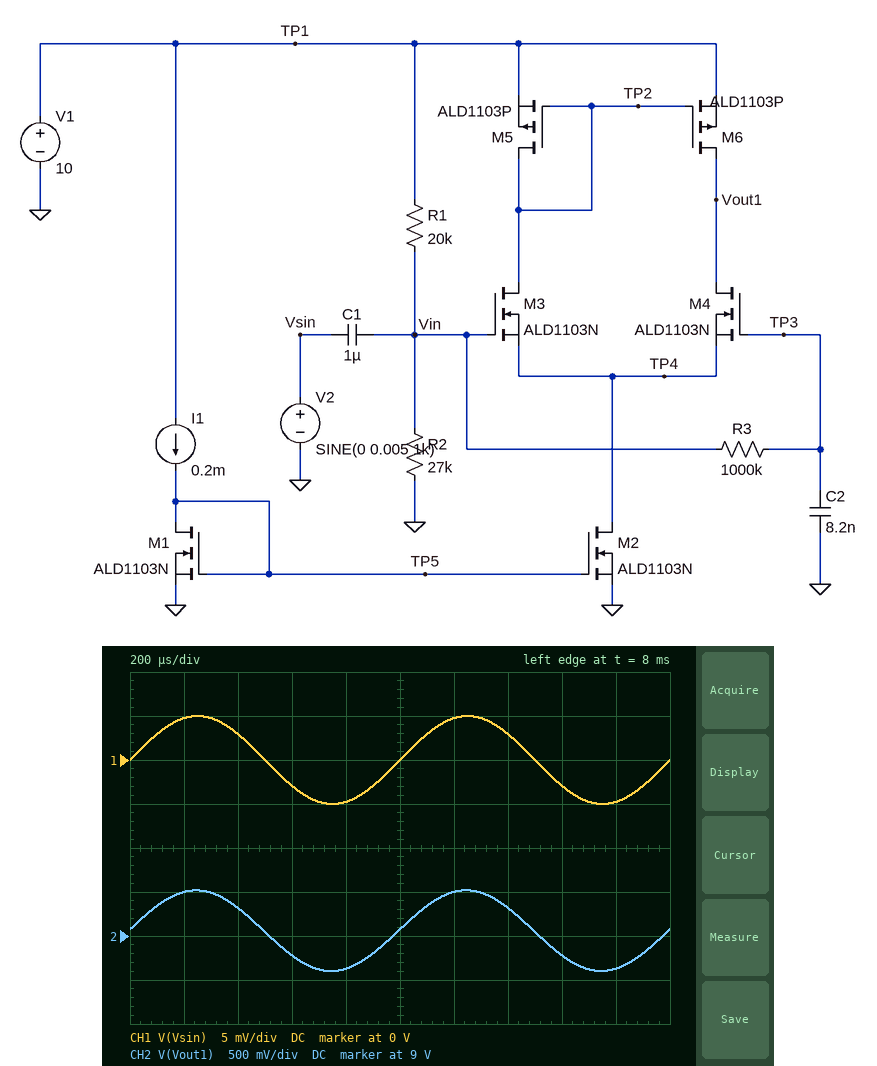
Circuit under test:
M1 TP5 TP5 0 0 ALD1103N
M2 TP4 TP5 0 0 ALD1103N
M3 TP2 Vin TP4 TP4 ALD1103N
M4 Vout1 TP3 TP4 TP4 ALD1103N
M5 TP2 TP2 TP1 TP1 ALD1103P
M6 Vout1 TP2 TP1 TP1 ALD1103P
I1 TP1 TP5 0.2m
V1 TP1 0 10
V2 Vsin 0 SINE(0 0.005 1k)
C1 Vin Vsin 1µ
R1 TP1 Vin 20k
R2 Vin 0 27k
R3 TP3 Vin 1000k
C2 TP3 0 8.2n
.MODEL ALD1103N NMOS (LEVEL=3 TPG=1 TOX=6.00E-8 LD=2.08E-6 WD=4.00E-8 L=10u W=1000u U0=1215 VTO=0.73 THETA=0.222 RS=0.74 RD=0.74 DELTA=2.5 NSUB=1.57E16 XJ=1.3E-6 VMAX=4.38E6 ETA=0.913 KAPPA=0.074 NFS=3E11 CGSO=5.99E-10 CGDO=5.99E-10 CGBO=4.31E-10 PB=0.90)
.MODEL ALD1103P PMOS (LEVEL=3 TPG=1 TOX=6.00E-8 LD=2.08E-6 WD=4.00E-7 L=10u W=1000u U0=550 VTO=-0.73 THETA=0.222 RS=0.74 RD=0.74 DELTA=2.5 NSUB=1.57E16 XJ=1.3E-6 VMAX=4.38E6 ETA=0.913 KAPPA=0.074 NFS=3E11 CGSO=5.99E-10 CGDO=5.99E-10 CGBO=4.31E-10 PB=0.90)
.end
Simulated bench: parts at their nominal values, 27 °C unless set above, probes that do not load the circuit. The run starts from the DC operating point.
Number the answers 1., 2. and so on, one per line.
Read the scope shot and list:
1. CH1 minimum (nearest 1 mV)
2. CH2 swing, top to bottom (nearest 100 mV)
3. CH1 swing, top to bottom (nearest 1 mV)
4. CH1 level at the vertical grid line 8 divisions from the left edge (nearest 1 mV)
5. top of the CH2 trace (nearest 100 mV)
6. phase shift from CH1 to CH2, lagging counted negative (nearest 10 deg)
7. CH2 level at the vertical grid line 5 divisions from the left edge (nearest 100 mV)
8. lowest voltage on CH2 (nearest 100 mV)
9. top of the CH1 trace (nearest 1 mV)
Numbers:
1. -5 mV
2. 900 mV
3. 10 mV
4. -3 mV
5. 9.5 V
6. 0 deg
7. 9.1 V
8. 8.6 V
9. 5 mV
